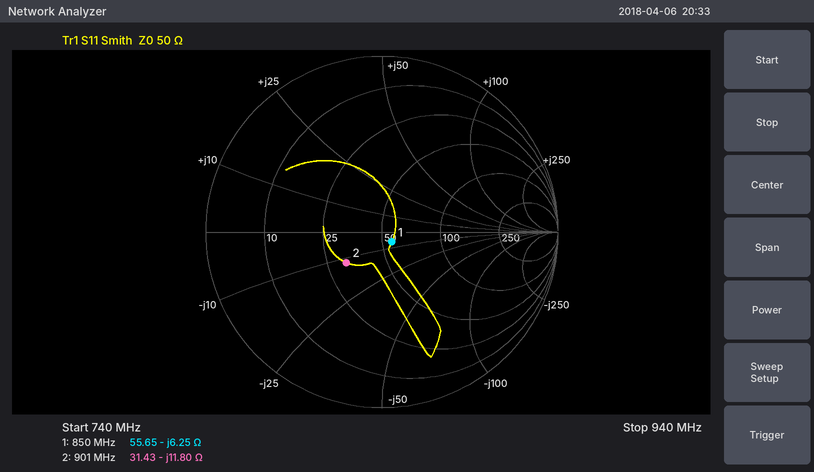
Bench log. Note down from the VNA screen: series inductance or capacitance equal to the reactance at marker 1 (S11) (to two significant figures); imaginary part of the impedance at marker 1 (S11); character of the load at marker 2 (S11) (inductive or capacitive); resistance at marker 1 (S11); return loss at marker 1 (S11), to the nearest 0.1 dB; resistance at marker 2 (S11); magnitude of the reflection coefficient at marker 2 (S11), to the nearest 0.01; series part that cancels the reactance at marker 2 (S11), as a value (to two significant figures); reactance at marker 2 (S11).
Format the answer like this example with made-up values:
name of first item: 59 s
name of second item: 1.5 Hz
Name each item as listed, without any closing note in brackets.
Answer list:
series inductance or capacitance equal to the reactance at marker 1 (S11): 30 pF
imaginary part of the impedance at marker 1: -6.25 Ω
character of the load at marker 2 (S11): capacitive
resistance at marker 1: 55.65 Ω
return loss at marker 1 (S11), to the nearest 0.1 dB: 22.0 dB
resistance at marker 2: 31.43 Ω
magnitude of the reflection coefficient at marker 2 (S11), to the nearest 0.01: 0.27
series part that cancels the reactance at marker 2 (S11), as a value: 2.1 nH
reactance at marker 2: -11.80 Ω
